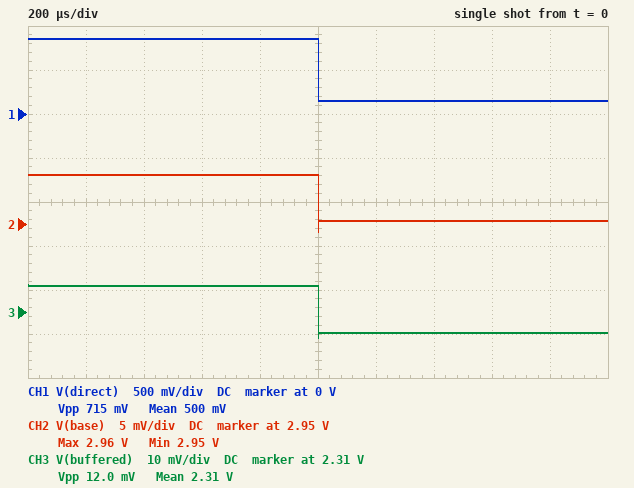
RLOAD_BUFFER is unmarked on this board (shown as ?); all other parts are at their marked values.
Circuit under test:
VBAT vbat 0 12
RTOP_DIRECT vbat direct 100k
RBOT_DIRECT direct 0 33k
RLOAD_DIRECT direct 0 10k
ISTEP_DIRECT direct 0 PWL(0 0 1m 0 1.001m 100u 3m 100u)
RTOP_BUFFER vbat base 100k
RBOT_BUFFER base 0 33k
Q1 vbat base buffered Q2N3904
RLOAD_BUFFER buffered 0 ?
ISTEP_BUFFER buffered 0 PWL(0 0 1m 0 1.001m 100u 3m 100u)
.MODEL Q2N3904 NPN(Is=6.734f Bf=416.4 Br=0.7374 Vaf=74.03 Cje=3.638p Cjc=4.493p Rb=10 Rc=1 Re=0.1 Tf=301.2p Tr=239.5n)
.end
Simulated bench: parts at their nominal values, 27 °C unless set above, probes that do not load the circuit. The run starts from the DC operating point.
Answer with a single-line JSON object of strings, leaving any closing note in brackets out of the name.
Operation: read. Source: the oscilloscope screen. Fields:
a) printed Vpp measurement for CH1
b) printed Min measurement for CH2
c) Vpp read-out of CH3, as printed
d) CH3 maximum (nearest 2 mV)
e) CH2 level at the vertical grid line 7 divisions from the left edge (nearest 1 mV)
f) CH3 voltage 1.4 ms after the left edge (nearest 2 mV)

{"printed Vpp measurement for CH1": "715 mV", "printed Min measurement for CH2": "2.95 V", "Vpp read-out of CH3, as printed": "12.0 mV", "CH3 maximum": "2.316 V", "CH2 level at the vertical grid line 7 divisions from the left edge": "2.950 V", "CH3 voltage 1.4 ms after the left edge": "2.306 V"}
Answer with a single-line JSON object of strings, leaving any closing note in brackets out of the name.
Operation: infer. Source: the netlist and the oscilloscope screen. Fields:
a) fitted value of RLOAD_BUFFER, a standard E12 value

{"fitted value of RLOAD_BUFFER, a standard E12 value": "5.6 kΩ"}
